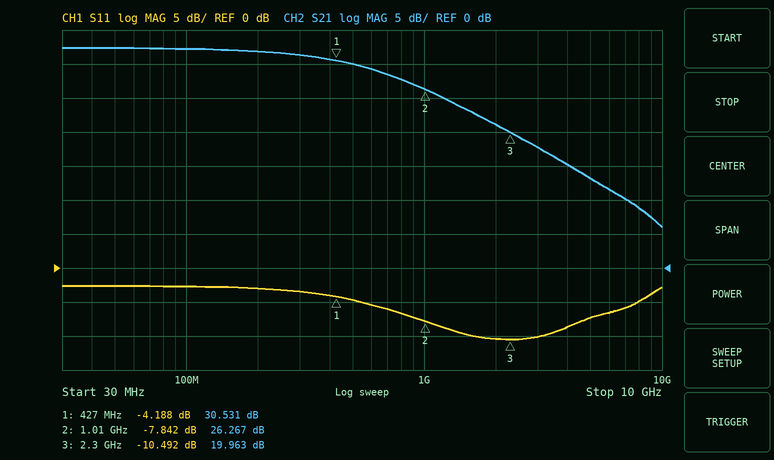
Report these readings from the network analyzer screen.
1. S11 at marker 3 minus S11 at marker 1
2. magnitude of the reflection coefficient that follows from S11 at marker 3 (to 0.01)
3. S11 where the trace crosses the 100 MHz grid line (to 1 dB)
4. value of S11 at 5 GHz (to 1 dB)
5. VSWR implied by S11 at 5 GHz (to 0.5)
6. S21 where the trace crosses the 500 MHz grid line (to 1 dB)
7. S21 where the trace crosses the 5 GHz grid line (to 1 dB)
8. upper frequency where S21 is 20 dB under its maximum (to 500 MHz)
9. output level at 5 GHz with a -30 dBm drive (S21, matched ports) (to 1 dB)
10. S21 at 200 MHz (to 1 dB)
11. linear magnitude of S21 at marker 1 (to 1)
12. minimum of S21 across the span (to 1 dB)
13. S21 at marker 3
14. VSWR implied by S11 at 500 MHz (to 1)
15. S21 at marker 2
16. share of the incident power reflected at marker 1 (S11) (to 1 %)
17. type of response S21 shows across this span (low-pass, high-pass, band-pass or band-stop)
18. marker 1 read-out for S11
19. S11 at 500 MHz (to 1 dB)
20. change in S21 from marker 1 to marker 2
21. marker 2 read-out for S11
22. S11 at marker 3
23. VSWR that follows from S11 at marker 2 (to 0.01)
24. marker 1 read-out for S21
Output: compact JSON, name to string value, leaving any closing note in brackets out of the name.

{"S11 at marker 3 minus S11 at marker 1": "-6.304 dB", "magnitude of the reflection coefficient that follows from S11 at marker 3": "0.30", "S11 where the trace crosses the 100 MHz grid line": "-3 dB", "value of S11 at 5 GHz": "-7 dB", "VSWR implied by S11 at 5 GHz": "2.5", "S21 where the trace crosses the 500 MHz grid line": "30 dB", "S21 where the trace crosses the 5 GHz grid line": "13 dB", "upper frequency where S21 is 20 dB under its maximum": "5.5 GHz", "output level at 5 GHz with a -30 dBm drive (S21, matched ports)": "-17 dBm", "S21 at 200 MHz": "32 dB", "linear magnitude of S21 at marker 1": "34", "minimum of S21 across the span": "6 dB", "S21 at marker 3": "19.963 dB", "VSWR implied by S11 at 500 MHz": "4", "S21 at marker 2": "26.267 dB", "share of the incident power reflected at marker 1 (S11)": "38 %", "type of response S21 shows across this span": "low-pass", "marker 1 read-out for S11": "-4.188 dB", "S11 at 500 MHz": "-5 dB", "change in S21 from marker 1 to marker 2": "-4.264 dB", "marker 2 read-out for S11": "-7.842 dB", "S11 at marker 3": "-10.492 dB", "VSWR that follows from S11 at marker 2": "2.36", "marker 1 read-out for S21": "30.531 dB"}
